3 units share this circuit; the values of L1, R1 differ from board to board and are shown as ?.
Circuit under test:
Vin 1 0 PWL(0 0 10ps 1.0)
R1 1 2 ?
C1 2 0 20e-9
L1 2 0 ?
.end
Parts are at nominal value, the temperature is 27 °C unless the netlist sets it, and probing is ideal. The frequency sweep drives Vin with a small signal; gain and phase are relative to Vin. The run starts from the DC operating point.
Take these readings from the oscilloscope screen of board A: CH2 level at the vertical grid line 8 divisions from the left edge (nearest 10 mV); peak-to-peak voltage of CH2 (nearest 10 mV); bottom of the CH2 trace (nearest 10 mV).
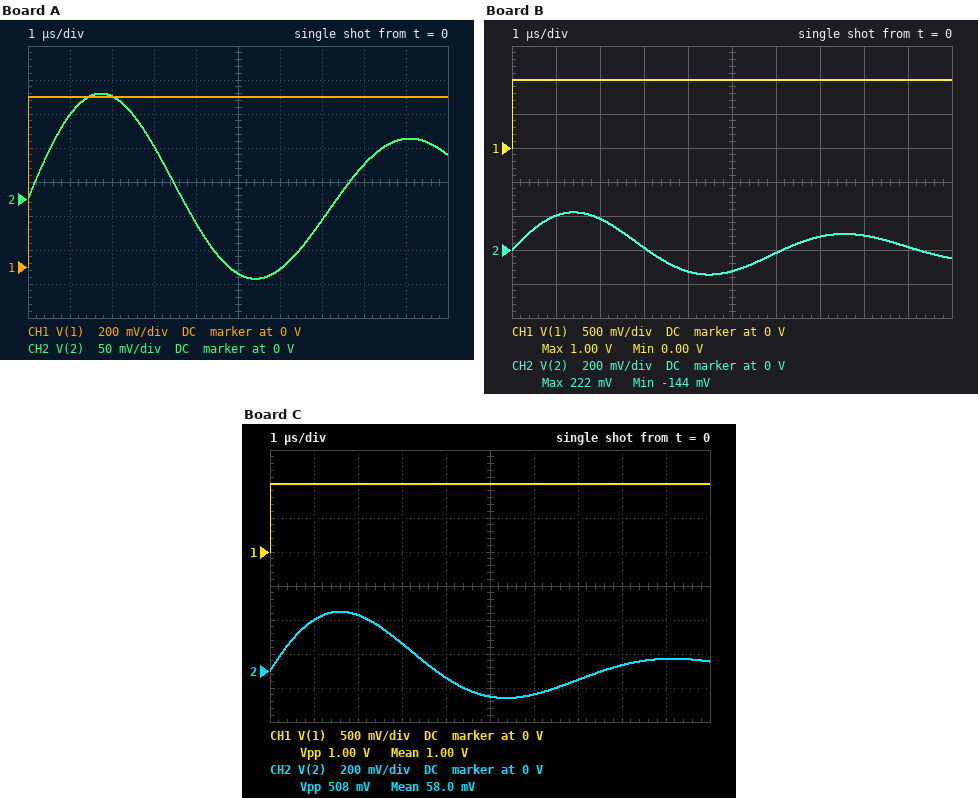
50 mV
270 mV
-120 mV
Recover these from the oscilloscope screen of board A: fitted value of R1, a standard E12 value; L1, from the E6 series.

330 Ω
68 µH
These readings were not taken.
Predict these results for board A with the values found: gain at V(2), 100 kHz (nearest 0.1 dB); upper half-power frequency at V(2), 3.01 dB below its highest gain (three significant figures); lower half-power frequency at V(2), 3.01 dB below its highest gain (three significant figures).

-11.4 dB
149 kHz
125 kHz
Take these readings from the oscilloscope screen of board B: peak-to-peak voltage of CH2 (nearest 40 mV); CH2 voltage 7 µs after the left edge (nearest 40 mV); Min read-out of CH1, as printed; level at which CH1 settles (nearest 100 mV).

360 mV
80 mV
0.00 V
1.0 V
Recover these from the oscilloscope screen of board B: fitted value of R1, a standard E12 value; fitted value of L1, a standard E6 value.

180 Ω
47 µH
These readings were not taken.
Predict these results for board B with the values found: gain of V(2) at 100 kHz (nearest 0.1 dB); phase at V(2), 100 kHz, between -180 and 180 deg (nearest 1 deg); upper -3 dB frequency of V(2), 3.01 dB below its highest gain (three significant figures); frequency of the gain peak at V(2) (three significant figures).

-12.0 dB
75 deg
188 kHz
164 kHz
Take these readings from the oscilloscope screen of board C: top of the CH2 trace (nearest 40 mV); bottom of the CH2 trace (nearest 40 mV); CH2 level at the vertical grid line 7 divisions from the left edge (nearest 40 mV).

360 mV
-160 mV
-40 mV
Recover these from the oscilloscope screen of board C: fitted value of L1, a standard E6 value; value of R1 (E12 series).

68 µH
120 Ω
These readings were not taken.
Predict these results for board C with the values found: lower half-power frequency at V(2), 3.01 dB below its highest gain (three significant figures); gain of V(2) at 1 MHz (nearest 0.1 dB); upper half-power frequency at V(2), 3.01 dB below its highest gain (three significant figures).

107 kHz
-23.4 dB
174 kHz
